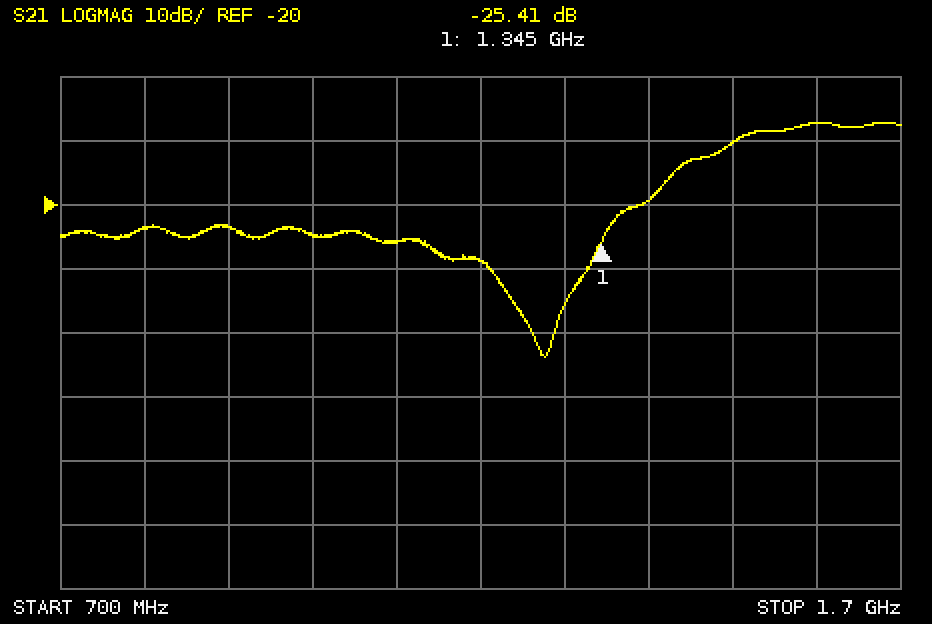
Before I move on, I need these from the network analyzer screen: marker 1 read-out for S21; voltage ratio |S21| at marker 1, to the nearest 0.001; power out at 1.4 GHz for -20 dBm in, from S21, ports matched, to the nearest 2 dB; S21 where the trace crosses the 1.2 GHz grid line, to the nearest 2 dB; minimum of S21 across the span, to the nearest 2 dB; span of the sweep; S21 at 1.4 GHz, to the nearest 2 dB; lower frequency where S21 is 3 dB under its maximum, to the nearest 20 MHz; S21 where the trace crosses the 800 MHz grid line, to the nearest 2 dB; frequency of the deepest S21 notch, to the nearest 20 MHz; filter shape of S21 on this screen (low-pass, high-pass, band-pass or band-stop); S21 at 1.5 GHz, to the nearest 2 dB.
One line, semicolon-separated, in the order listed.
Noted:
-25.41 dB; 0.054; -40 dBm; -28 dB; -44 dB; 1 GHz; -20 dB; 1.50 GHz; -24 dB; 1.28 GHz; high-pass; -10 dB
